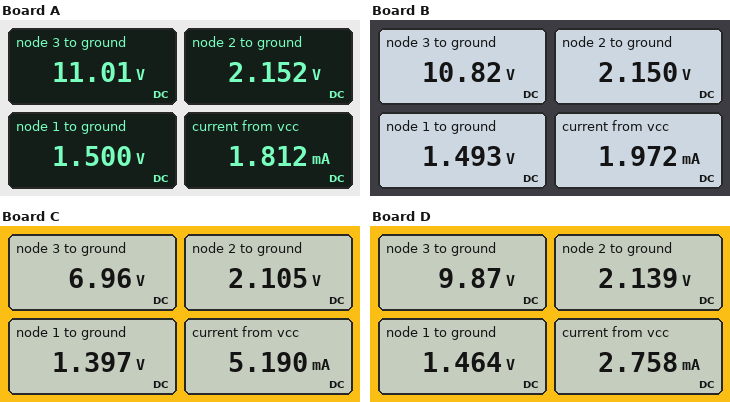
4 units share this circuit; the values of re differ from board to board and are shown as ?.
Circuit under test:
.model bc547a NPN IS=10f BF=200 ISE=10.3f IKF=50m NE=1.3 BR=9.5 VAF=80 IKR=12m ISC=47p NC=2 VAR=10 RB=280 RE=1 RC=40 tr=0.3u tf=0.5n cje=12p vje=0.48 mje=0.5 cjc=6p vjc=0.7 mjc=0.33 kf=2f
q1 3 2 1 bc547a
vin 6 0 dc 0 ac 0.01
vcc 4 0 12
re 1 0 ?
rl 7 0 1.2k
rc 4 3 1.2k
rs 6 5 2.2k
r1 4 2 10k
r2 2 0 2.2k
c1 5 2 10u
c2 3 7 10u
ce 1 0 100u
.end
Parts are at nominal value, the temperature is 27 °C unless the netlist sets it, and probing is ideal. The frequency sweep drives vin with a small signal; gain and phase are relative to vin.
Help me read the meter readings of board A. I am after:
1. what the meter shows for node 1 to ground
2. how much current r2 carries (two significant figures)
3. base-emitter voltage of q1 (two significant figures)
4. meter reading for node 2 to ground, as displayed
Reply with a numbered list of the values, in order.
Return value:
1. 1.500 V
2. 980 µA
3. 650 mV
4. 2.152 V
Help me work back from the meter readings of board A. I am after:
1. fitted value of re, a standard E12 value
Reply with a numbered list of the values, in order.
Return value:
1. 1.8 kΩ
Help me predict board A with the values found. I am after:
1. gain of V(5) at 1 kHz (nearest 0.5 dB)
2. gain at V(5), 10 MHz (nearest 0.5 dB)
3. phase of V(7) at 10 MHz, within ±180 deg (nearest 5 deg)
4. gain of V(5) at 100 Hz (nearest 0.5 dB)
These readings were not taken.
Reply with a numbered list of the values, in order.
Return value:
1. -8.5 dB
2. -18.5 dB
3. 95 deg
4. -8.0 dB
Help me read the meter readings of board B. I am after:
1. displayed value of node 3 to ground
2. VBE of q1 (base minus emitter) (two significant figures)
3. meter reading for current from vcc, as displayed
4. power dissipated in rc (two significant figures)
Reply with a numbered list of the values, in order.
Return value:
1. 10.82 V
2. 660 mV
3. 1.972 mA
4. 1.2 mW
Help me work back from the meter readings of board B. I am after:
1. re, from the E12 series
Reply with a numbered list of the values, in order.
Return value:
1. 1.5 kΩ
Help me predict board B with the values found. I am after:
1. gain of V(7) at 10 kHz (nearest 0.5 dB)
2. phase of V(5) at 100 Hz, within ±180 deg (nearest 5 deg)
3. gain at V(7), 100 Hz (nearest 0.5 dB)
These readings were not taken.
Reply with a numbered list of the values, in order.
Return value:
1. 17.0 dB
2. -10 deg
3. 16.5 dB
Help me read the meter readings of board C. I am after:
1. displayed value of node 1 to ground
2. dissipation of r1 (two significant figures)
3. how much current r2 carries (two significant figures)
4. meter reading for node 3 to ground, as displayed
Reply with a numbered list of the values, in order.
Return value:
1. 1.397 V
2. 9.8 mW
3. 960 µA
4. 6.96 V
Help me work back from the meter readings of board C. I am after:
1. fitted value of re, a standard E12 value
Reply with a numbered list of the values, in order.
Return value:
1. 330 Ω
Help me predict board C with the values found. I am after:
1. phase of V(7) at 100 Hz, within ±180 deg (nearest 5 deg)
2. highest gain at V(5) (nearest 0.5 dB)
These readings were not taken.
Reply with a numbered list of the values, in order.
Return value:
1. -135 deg
2. 0 dB
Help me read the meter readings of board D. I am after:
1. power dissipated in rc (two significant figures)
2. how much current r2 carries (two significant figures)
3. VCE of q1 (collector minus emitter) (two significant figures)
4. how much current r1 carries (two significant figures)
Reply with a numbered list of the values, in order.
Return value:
1. 3.8 mW
2. 970 µA
3. 8.4 V
4. 990 µA
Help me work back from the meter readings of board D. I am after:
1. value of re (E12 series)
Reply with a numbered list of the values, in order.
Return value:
1. 820 Ω
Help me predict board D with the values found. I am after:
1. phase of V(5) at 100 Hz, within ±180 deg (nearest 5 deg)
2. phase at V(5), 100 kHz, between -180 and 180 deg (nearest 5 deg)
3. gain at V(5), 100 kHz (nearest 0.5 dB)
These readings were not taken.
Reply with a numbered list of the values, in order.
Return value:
1. -15 deg
2. -5 deg
3. -10.0 dB
